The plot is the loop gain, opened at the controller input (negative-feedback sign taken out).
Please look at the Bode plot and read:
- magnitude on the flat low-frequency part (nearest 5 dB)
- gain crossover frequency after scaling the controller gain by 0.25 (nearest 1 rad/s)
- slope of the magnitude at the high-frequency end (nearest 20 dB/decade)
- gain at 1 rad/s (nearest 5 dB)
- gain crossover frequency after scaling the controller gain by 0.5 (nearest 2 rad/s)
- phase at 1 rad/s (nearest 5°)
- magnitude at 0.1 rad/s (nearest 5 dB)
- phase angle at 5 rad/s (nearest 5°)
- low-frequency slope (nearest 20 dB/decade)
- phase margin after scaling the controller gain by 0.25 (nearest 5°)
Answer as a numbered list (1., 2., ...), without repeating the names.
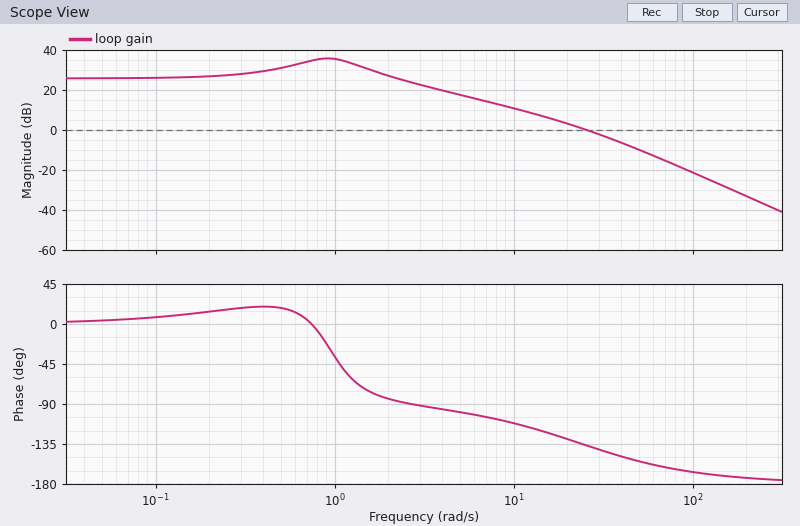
1. 25 dB
2. 9 rad/s
3. -40 dB/decade
4. 35 dB
5. 16 rad/s
6. -35°
7. 25 dB
8. -100°
9. 0 dB/decade
10. 70°
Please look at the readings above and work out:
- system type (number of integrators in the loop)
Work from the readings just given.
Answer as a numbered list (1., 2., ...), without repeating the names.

1. 0
